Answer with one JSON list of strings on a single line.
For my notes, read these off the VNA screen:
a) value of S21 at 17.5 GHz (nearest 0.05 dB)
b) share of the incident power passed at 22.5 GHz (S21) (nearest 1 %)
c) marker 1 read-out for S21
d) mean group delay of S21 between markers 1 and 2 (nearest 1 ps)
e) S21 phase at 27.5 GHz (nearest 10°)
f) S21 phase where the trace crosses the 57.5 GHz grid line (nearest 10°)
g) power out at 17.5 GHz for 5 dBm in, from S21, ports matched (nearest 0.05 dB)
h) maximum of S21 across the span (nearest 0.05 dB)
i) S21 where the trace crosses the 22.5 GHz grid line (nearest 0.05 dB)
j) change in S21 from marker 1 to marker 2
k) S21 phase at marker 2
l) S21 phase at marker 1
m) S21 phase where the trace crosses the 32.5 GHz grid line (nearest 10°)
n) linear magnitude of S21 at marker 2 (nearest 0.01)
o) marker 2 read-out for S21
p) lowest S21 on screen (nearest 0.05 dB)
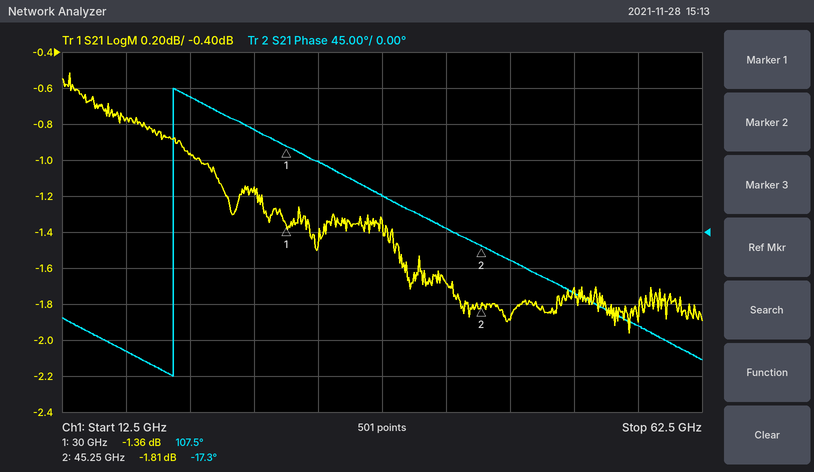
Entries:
["-0.75 dB", "80 %", "-1.36 dB", "23 ps", "130°", "-120°", "4.25 dBm", "-0.50 dB", "-0.95 dB", "-0.45 dB", "-17.3°", "107.5°", "90°", "0.81", "-1.81 dB", "-1.95 dB"]
